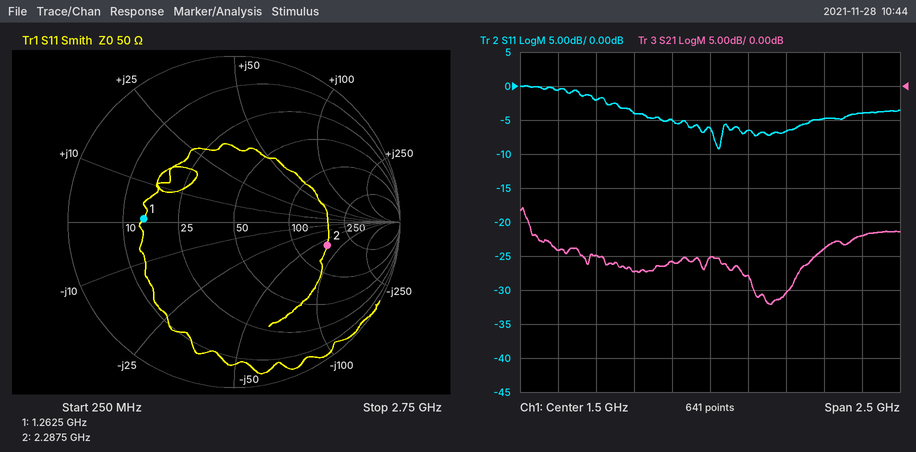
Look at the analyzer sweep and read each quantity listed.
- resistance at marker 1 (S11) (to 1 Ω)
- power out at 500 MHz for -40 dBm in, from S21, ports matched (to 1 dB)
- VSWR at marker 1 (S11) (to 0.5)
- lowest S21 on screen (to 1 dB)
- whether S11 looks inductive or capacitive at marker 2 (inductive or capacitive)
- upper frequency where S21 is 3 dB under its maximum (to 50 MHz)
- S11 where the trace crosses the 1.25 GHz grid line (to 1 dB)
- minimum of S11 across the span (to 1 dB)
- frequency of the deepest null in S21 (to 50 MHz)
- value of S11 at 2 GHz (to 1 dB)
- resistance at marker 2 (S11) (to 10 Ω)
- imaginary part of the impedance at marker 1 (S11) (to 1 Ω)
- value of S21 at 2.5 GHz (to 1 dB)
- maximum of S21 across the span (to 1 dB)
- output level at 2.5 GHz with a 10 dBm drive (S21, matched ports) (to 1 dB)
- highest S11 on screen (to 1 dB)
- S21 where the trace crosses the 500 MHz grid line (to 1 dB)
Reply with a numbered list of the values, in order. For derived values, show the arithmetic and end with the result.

1. 15 Ω
2. -40 dBm + (-24 dB) = -64 dBm
3. 3.5
4. -32 dB
5. capacitive
6. 300 MHz
7. -5 dB
8. -9 dB
9. 1.90 GHz
10. -7 dB
11. 160 Ω
12. +1 Ω
13. -22 dB
14. -18 dB
15. 10 dBm + (-22 dB) = -12 dBm
16. 0 dB
17. -24 dB
